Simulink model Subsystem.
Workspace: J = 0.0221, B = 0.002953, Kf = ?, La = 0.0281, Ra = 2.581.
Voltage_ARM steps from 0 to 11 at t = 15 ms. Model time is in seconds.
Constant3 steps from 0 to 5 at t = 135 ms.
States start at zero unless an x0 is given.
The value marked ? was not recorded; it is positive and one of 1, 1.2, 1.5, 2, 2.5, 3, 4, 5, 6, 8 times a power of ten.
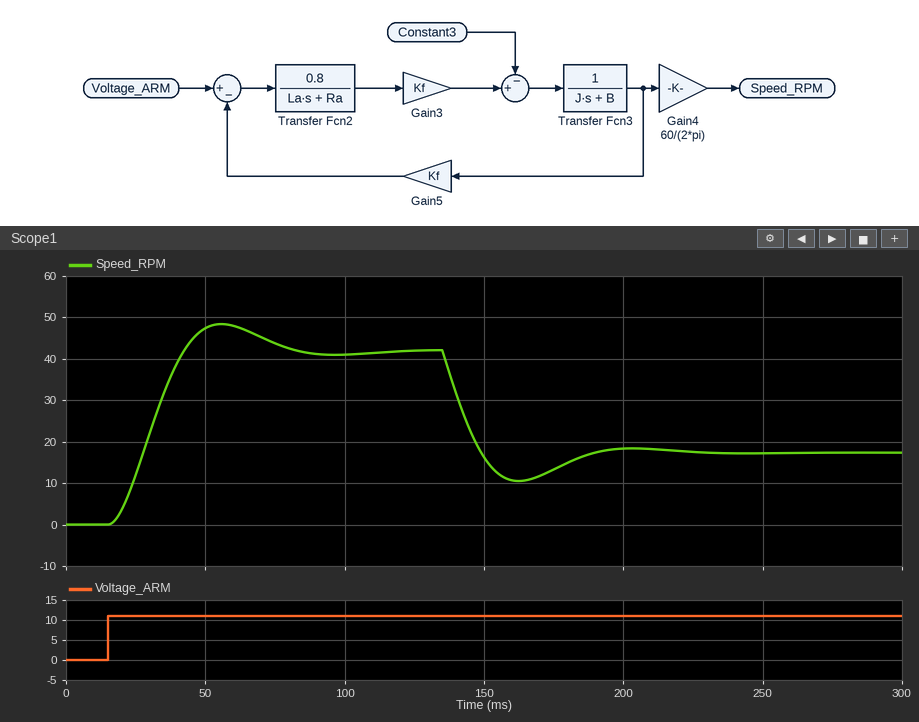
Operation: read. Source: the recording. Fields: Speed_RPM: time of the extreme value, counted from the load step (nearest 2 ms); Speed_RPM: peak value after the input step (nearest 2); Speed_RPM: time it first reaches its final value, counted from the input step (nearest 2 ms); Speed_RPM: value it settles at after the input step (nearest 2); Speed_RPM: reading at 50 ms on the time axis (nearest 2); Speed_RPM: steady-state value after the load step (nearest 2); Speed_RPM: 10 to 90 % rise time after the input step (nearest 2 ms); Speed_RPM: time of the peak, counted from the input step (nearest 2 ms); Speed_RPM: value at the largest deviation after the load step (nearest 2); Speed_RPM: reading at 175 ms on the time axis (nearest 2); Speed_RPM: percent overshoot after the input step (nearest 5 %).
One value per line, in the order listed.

28 ms
48
28 ms
42
48
18
18 ms
40 ms
10
14
15 %
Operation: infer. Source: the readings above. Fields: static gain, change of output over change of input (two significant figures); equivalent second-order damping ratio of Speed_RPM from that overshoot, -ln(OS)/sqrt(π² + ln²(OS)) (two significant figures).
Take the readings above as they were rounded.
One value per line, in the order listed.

3.8
0.52
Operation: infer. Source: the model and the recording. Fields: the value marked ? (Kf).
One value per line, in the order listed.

2.5
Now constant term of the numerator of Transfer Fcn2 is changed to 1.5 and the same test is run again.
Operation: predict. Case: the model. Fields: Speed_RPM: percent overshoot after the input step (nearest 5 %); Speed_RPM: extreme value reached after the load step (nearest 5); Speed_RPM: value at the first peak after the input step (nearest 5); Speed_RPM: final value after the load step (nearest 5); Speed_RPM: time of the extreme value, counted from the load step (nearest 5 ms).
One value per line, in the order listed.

30 %
20
55
30
15 ms
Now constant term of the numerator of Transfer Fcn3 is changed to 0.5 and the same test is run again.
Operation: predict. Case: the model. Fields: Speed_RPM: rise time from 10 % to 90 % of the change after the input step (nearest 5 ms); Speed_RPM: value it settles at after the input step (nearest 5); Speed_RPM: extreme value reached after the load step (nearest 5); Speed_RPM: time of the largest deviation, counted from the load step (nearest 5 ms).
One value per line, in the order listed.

35 ms
40
15
55 ms
